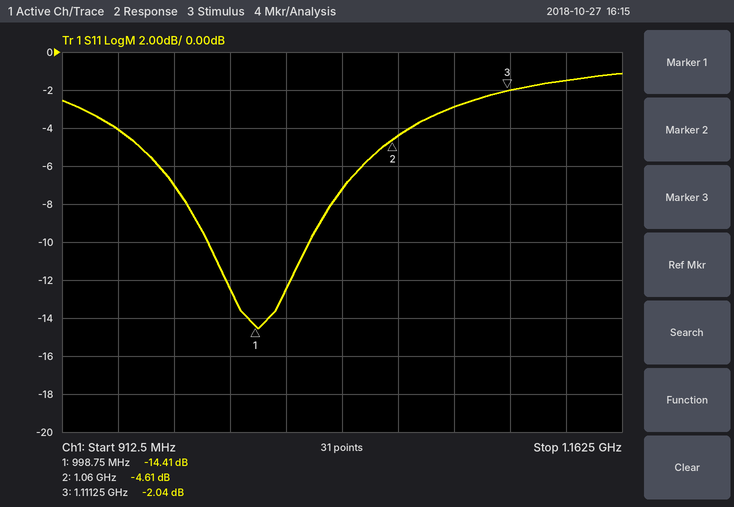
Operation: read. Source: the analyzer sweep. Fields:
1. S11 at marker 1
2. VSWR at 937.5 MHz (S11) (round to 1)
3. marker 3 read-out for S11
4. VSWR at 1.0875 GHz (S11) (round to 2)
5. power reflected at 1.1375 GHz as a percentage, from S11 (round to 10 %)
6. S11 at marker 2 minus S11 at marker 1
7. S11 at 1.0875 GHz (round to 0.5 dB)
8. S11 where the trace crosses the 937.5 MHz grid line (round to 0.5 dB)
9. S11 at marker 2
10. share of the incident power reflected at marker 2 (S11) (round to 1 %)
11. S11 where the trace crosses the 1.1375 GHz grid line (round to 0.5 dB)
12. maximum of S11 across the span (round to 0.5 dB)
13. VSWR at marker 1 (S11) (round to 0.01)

-14.41 dB
4
-2.04 dB
6
70 %
9.80 dB
-3.0 dB
-4.0 dB
-4.61 dB
35 %
-1.5 dB
-1.0 dB
1.47
